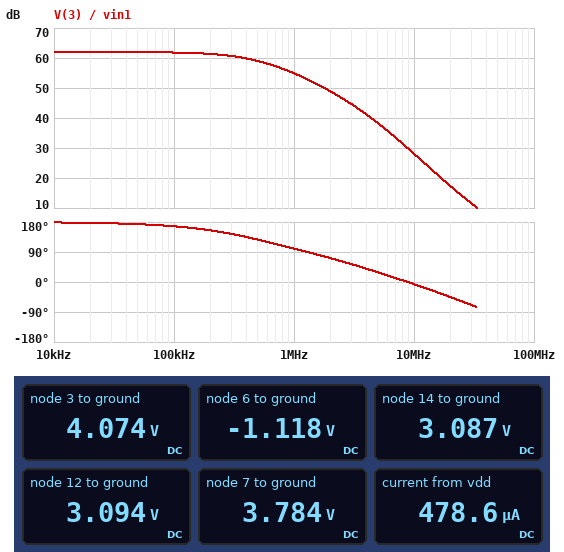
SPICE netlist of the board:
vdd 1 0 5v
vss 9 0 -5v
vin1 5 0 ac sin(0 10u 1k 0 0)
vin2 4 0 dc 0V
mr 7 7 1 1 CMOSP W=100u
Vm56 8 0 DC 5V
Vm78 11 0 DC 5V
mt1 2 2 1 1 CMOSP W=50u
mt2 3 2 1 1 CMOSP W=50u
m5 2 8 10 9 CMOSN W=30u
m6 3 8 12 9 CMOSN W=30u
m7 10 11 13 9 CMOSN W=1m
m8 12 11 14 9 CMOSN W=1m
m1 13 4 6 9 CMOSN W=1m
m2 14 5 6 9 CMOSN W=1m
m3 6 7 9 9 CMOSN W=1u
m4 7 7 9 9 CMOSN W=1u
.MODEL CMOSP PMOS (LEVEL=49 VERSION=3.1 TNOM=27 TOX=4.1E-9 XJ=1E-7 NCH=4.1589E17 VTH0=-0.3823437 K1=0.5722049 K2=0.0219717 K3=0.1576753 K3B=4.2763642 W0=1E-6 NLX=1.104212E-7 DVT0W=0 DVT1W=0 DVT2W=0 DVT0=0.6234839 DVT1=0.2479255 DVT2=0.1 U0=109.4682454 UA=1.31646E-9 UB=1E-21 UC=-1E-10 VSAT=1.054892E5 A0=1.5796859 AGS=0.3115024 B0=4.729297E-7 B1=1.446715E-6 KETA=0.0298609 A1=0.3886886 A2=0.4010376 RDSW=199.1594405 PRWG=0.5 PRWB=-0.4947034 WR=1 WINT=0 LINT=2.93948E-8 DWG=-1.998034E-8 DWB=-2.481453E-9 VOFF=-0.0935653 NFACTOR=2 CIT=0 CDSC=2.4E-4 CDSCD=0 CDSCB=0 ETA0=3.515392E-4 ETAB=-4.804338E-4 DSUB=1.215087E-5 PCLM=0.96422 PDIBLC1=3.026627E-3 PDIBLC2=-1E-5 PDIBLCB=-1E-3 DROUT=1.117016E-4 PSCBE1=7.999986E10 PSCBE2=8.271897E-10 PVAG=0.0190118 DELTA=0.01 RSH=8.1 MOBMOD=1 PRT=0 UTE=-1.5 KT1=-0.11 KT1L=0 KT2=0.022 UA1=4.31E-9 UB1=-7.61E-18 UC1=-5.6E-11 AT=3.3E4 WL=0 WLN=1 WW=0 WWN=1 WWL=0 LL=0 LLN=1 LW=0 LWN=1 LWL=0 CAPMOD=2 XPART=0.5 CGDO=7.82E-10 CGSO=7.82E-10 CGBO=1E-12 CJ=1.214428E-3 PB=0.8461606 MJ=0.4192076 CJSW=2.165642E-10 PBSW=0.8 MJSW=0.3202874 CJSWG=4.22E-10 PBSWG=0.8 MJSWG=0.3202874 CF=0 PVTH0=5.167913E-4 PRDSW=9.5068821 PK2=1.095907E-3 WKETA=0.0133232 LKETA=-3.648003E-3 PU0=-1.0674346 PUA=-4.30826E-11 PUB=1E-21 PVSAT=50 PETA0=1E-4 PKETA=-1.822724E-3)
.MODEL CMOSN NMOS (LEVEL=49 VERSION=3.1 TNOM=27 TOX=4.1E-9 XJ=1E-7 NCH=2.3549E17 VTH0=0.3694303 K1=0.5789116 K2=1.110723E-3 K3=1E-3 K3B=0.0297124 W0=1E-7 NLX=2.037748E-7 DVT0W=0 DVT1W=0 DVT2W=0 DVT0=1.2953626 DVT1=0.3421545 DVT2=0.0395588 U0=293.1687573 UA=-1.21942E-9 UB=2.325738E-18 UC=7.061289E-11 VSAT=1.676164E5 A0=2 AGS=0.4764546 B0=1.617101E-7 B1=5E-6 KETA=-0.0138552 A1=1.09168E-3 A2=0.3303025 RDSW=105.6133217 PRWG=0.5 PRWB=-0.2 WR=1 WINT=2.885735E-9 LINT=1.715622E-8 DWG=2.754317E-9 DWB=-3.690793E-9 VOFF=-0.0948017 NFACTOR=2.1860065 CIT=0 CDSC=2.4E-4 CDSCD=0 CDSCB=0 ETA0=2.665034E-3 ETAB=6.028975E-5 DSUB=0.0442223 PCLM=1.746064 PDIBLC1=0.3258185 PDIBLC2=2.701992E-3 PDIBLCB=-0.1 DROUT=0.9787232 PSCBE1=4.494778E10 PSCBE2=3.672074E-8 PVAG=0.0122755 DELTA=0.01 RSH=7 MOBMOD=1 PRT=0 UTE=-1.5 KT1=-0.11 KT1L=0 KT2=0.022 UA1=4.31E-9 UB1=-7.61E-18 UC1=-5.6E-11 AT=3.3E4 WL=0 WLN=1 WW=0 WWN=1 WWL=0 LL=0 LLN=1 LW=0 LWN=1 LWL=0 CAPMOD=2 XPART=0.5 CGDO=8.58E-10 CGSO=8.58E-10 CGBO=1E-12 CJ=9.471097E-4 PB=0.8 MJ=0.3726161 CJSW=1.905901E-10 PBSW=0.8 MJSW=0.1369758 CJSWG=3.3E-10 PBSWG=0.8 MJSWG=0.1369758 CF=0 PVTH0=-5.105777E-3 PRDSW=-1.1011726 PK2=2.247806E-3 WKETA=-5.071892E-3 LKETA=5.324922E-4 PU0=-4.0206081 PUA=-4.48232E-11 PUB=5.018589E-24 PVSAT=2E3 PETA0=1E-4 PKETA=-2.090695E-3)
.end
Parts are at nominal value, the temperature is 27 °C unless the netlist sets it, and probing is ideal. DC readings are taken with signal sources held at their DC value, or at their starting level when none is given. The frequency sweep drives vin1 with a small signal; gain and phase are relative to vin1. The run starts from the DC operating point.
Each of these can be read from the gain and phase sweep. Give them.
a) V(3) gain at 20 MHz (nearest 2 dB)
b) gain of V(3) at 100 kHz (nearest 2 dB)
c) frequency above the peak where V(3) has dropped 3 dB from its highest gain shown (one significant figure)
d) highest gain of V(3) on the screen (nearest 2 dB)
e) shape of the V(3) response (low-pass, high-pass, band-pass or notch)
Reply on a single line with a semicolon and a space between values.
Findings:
18 dB; 62 dB; 500 kHz; 62 dB; low-pass
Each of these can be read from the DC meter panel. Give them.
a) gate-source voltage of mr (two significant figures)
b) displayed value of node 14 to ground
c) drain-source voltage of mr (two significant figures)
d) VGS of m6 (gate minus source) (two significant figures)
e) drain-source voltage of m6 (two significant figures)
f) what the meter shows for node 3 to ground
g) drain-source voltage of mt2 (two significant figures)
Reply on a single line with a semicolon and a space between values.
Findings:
-1.2 V; 3.087 V; -1.2 V; 1.9 V; 980 mV; 4.074 V; -930 mV
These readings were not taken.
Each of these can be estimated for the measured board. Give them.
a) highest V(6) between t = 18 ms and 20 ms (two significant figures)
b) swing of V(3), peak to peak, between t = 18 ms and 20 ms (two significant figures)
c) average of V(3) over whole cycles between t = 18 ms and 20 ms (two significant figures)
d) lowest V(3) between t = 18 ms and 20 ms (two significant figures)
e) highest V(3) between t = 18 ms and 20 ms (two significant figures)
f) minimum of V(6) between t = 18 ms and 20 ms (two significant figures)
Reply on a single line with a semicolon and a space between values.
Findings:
-1.1 V; 25 mV; 4.1 V; 4.1 V; 4.1 V; -1.1 V
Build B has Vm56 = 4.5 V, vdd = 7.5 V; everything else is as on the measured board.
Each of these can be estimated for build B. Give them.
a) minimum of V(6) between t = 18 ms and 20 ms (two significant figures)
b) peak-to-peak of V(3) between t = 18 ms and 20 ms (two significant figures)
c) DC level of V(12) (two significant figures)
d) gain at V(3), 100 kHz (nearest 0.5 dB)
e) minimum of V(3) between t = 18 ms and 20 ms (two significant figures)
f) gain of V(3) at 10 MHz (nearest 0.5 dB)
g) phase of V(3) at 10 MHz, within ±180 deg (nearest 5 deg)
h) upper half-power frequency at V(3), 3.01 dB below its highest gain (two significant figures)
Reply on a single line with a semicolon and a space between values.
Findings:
-1.1 V; 24 mV; 2.7 V; 61.5 dB; 6.6 V; 26.0 dB; -10 deg; 490 kHz
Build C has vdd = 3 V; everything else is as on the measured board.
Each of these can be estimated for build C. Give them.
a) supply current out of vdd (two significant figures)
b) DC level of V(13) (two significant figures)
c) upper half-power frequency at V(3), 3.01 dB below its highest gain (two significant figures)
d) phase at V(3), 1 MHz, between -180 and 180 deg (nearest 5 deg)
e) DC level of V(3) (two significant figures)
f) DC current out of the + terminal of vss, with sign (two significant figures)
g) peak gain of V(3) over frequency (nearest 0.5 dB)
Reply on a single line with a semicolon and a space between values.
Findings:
510 µA; 1.9 V; 17 kHz; 75 deg; 2.0 V; -510 µA; 51.5 dB
